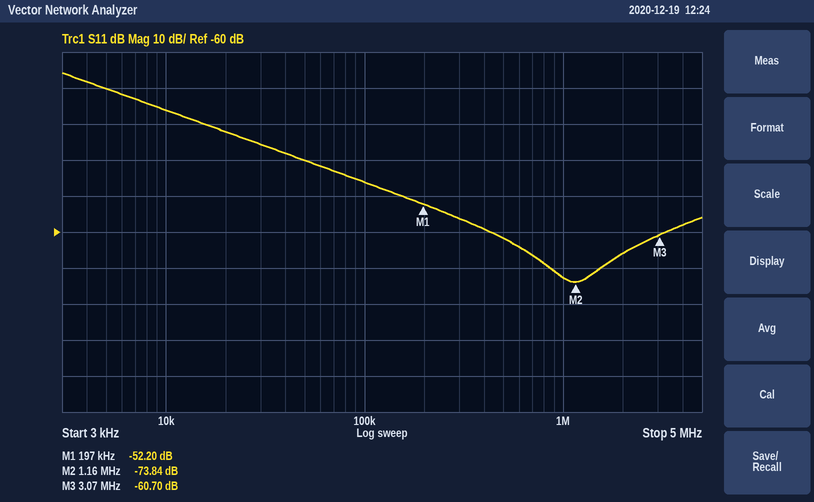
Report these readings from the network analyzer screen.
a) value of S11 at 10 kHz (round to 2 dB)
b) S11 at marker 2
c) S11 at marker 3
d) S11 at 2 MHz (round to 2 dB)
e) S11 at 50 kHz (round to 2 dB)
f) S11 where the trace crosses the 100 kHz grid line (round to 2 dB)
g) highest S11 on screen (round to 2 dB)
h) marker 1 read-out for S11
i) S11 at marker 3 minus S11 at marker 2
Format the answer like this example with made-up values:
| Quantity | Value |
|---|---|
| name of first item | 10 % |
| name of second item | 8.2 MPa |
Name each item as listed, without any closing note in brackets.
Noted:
| Quantity | Value |
|---|---|
| value of S11 at 10 kHz | -26 dB |
| S11 at marker 2 | -73.84 dB |
| S11 at marker 3 | -60.70 dB |
| S11 at 2 MHz | -66 dB |
| S11 at 50 kHz | -40 dB |
| S11 where the trace crosses the 100 kHz grid line | -46 dB |
| highest S11 on screen | -16 dB |
| marker 1 read-out for S11 | -52.20 dB |
| S11 at marker 3 minus S11 at marker 2 | 13.14 dB |
